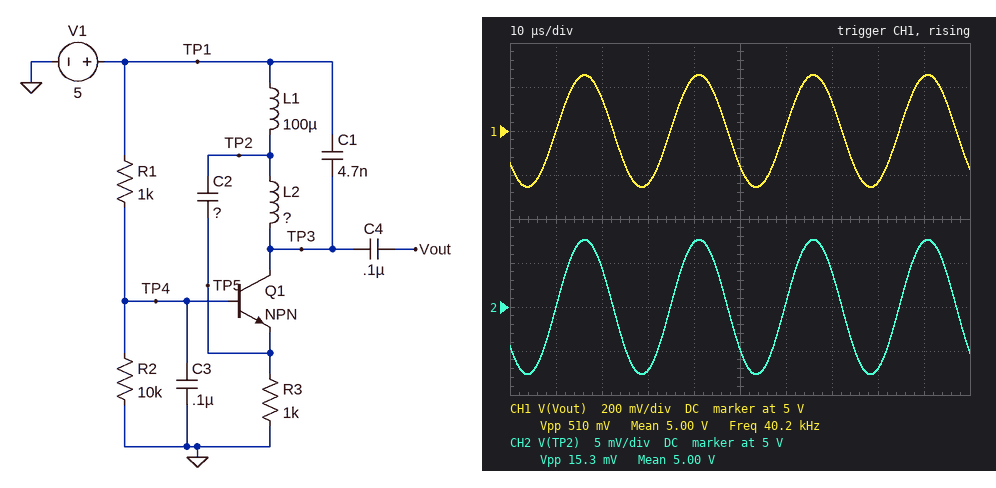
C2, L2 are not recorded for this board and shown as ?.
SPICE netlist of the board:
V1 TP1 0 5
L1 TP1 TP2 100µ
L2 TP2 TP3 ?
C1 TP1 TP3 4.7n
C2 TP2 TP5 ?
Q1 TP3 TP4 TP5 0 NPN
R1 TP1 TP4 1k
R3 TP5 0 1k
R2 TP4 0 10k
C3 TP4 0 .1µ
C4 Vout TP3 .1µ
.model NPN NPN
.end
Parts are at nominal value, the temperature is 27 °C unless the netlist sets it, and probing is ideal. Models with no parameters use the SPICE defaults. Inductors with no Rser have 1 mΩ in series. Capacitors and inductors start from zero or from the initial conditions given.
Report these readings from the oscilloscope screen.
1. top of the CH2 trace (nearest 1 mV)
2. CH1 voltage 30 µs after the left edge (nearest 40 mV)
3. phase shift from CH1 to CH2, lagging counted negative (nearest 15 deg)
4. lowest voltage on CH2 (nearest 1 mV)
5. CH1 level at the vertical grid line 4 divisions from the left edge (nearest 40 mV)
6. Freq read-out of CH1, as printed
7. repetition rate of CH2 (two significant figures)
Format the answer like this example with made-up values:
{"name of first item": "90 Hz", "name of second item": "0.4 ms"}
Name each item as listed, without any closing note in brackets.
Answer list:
{"top of the CH2 trace": "5.008 V", "CH1 voltage 30 µs after the left edge": "4.76 V", "phase shift from CH1 to CH2, lagging counted negative": "0 deg", "lowest voltage on CH2": "4.992 V", "CH1 level at the vertical grid line 4 divisions from the left edge": "5.24 V", "Freq read-out of CH1, as printed": "40.2 kHz", "repetition rate of CH2": "40 kHz"}
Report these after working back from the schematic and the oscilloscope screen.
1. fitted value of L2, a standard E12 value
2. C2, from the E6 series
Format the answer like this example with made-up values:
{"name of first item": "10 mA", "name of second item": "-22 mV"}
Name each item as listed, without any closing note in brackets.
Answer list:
{"fitted value of L2, a standard E12 value": "3.3 mH", "C2, from the E6 series": "3.3 nF"}
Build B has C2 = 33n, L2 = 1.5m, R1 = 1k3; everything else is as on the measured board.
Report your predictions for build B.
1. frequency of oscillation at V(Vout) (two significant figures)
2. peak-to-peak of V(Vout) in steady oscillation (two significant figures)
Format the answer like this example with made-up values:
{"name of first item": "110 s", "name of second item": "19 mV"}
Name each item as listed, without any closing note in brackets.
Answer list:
{"frequency of oscillation at V(Vout)": "62 kHz", "peak-to-peak of V(Vout) in steady oscillation": "6.6 V"}
